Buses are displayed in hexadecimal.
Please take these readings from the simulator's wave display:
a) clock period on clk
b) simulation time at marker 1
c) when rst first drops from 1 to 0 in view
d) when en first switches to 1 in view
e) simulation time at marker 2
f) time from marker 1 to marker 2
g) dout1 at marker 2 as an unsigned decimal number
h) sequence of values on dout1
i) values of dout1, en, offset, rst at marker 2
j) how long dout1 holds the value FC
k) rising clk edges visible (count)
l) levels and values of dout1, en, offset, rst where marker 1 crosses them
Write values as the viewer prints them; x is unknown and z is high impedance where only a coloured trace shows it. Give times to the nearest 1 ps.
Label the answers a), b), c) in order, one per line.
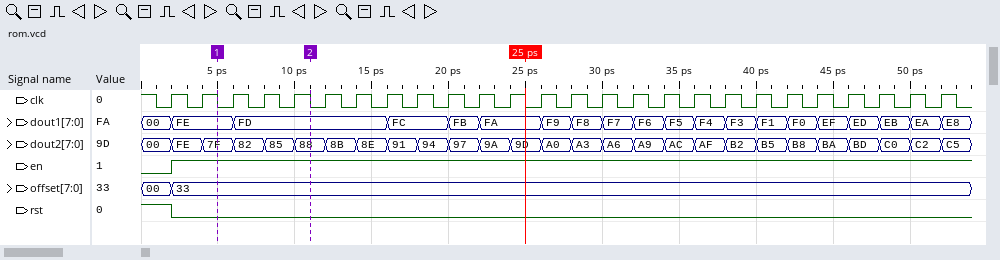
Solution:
a) 2 ps
b) 5 ps
c) 2 ps
d) 2 ps
e) 11 ps
f) 6 ps
g) 253
h) 00, FE, FD, FC, FB, FA, F9, F8, F7, F6, F5, F4, F3, F1, F0, EF, ED, EB, EA, E8
i) dout1=FD, en=1, offset=33, rst=0
j) 4 ps
k) 26
l) dout1=FE, en=1, offset=33, rst=0
